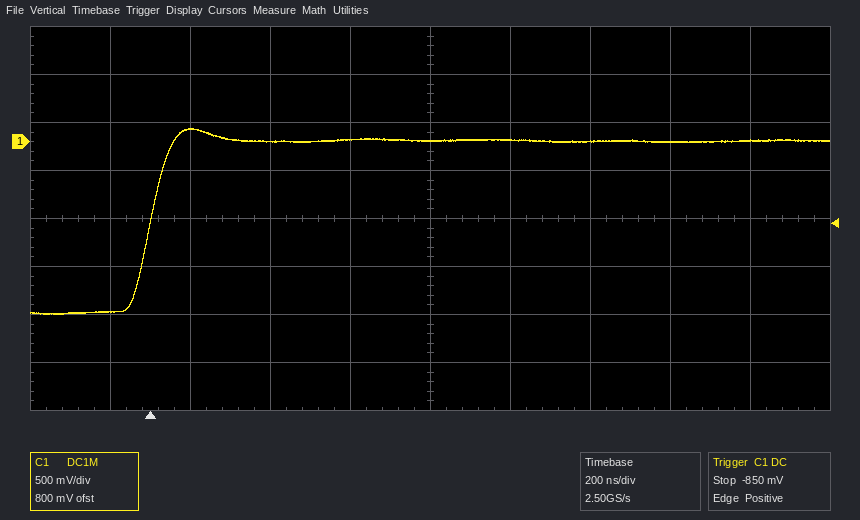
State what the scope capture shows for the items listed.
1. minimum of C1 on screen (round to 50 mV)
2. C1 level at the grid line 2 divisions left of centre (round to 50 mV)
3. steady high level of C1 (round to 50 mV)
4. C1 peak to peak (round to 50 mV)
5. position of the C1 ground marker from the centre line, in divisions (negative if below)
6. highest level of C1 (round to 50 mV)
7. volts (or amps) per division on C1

-1.80 V
0 mV
0 mV
1.95 V
+1.6 div
150 mV
500 mV
